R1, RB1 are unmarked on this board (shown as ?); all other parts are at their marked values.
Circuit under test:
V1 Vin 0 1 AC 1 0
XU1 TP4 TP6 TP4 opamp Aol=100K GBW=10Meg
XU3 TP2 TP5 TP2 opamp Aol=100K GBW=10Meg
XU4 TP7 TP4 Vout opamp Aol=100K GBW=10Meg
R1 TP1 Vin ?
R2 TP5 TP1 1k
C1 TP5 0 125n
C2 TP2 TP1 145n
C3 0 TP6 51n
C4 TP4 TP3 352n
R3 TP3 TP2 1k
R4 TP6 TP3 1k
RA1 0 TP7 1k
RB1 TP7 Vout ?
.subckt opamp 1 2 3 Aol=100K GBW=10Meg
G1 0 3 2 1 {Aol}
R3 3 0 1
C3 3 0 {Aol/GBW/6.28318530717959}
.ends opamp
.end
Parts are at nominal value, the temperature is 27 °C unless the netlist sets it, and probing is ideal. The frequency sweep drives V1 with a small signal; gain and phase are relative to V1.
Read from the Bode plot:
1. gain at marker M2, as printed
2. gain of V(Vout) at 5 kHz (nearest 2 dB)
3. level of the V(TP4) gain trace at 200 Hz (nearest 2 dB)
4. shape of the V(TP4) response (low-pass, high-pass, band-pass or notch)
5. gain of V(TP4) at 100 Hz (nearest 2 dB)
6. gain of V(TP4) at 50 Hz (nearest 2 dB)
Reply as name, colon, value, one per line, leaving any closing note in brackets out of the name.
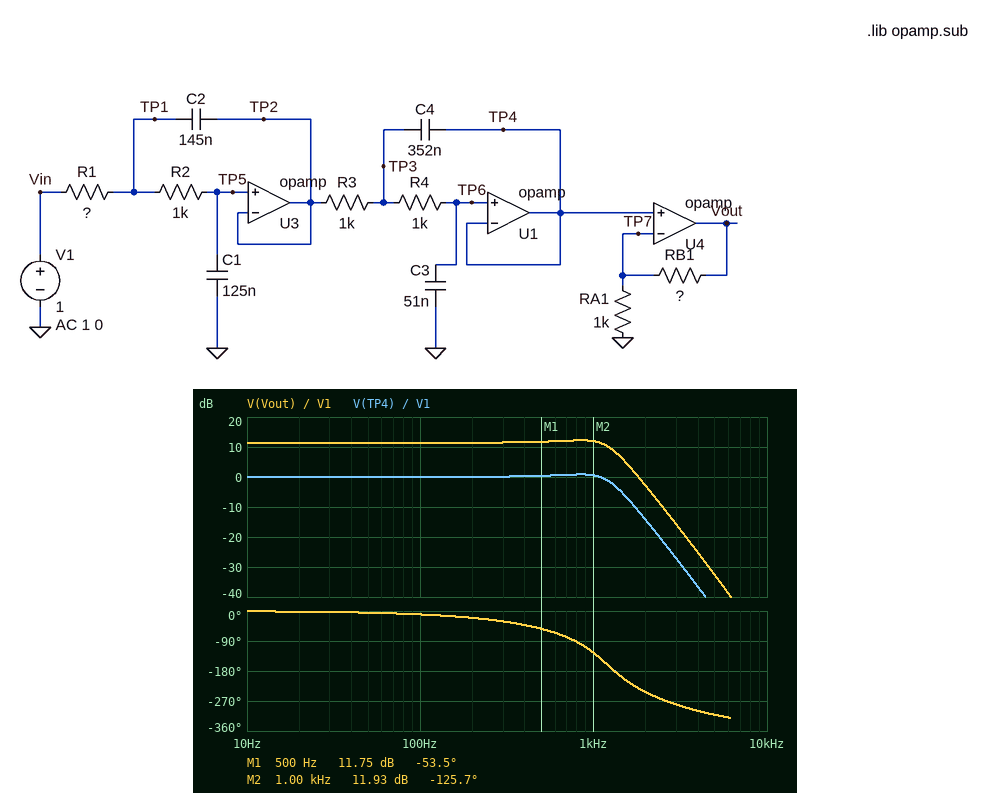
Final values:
gain at marker M2, as printed: 11.93 dB
gain of V(Vout) at 5 kHz: -32 dB
level of the V(TP4) gain trace at 200 Hz: 0 dB
shape of the V(TP4) response: low-pass
gain of V(TP4) at 100 Hz: 0 dB
gain of V(TP4) at 50 Hz: 0 dB
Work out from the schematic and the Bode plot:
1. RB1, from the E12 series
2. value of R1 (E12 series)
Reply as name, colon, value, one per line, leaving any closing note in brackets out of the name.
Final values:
RB1, from the E12 series: 2.7 kΩ
value of R1: 470 Ω
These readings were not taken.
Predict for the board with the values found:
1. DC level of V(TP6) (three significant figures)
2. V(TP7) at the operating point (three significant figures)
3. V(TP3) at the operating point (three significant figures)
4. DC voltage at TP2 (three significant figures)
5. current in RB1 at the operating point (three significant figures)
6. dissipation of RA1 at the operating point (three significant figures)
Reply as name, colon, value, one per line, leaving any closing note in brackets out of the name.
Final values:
DC level of V(TP6): 1.00 V
V(TP7) at the operating point: 1.00 V
V(TP3) at the operating point: 1.00 V
DC voltage at TP2: 1.00 V
current in RB1 at the operating point: 1.00 mA
dissipation of RA1 at the operating point: 1.00 mW
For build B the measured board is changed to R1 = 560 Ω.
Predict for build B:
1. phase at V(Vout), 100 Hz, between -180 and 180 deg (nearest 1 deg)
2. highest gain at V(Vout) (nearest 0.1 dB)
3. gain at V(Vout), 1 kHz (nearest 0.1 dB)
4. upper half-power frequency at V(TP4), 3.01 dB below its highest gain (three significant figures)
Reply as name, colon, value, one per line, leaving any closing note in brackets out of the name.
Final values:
phase at V(Vout), 100 Hz, between -180 and 180 deg: -11 deg
highest gain at V(Vout): 12.1 dB
gain at V(Vout), 1 kHz: 11.7 dB
upper half-power frequency at V(TP4), 3.01 dB below its highest gain: 1.26 kHz
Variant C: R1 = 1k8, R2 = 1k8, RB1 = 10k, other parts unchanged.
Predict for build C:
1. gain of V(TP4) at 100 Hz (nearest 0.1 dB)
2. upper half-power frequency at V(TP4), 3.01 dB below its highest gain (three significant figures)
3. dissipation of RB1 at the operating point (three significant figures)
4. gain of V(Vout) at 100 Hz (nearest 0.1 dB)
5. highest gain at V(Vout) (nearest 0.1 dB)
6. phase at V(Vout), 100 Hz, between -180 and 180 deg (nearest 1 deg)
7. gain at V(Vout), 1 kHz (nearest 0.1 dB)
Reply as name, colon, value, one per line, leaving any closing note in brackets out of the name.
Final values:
gain of V(TP4) at 100 Hz: -0.1 dB
upper half-power frequency at V(TP4), 3.01 dB below its highest gain: 589 Hz
dissipation of RB1 at the operating point: 10.0 mW
gain of V(Vout) at 100 Hz: 20.7 dB
highest gain at V(Vout): 20.8 dB
phase at V(Vout), 100 Hz, between -180 and 180 deg: -20 deg
gain at V(Vout), 1 kHz: 14.0 dB
